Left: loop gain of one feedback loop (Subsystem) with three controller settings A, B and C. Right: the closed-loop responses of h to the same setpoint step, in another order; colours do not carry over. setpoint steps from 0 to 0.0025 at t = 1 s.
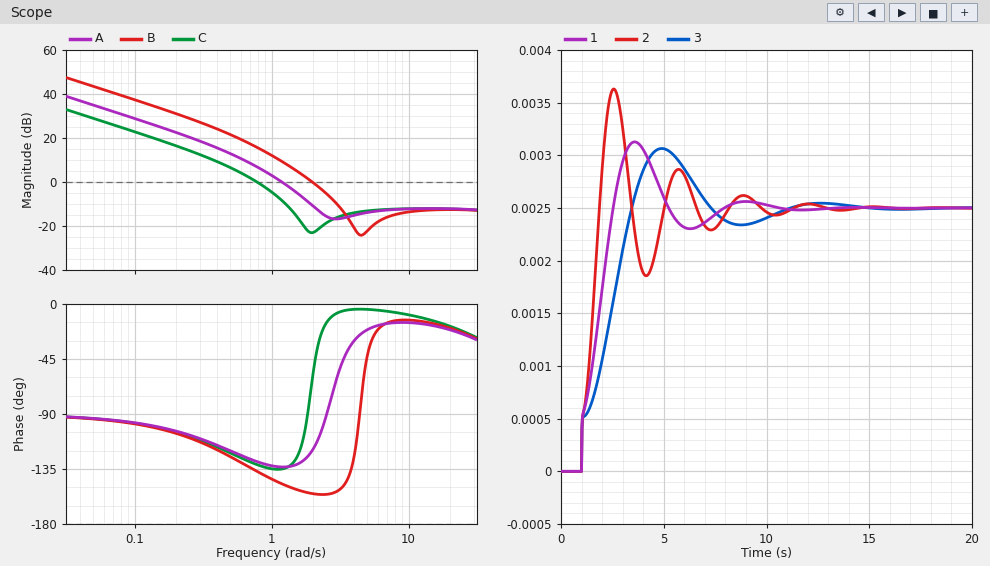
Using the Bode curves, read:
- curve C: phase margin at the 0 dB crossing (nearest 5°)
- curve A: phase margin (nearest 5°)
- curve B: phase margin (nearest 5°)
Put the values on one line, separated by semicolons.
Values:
50°; 45°; 25°
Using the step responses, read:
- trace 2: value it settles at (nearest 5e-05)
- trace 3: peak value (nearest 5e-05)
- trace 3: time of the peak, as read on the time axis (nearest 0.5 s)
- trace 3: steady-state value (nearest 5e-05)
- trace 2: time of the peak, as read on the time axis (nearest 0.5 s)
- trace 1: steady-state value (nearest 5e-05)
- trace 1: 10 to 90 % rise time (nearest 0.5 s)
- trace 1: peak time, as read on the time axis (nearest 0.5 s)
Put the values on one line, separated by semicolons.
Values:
0.00250; 0.00305; 5.0 s; 0.00250; 2.5 s; 0.00250; 1.5 s; 3.5 s
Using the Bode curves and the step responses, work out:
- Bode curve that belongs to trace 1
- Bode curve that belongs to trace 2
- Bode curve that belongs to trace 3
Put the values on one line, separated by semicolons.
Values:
A; B; C
